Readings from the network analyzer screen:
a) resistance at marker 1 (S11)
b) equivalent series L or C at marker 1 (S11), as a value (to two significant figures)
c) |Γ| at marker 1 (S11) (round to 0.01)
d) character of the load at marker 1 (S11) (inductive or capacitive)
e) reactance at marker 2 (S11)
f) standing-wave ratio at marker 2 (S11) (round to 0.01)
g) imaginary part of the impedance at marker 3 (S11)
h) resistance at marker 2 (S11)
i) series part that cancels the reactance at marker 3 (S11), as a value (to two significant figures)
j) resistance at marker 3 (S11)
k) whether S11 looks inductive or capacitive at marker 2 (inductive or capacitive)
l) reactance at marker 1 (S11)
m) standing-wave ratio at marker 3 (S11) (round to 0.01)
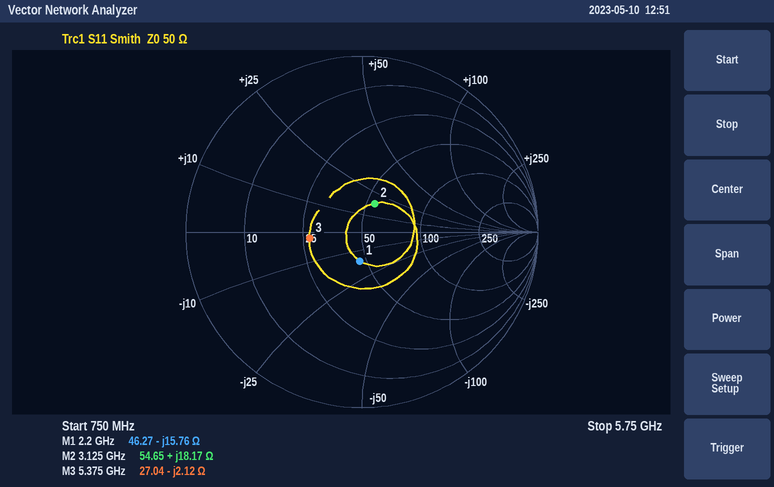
46.27 Ω
4.6 pF
0.17
capacitive
+18.17 Ω
1.43
-2.12 Ω
54.65 Ω
63 pH
27.04 Ω
inductive
-15.76 Ω
1.85
